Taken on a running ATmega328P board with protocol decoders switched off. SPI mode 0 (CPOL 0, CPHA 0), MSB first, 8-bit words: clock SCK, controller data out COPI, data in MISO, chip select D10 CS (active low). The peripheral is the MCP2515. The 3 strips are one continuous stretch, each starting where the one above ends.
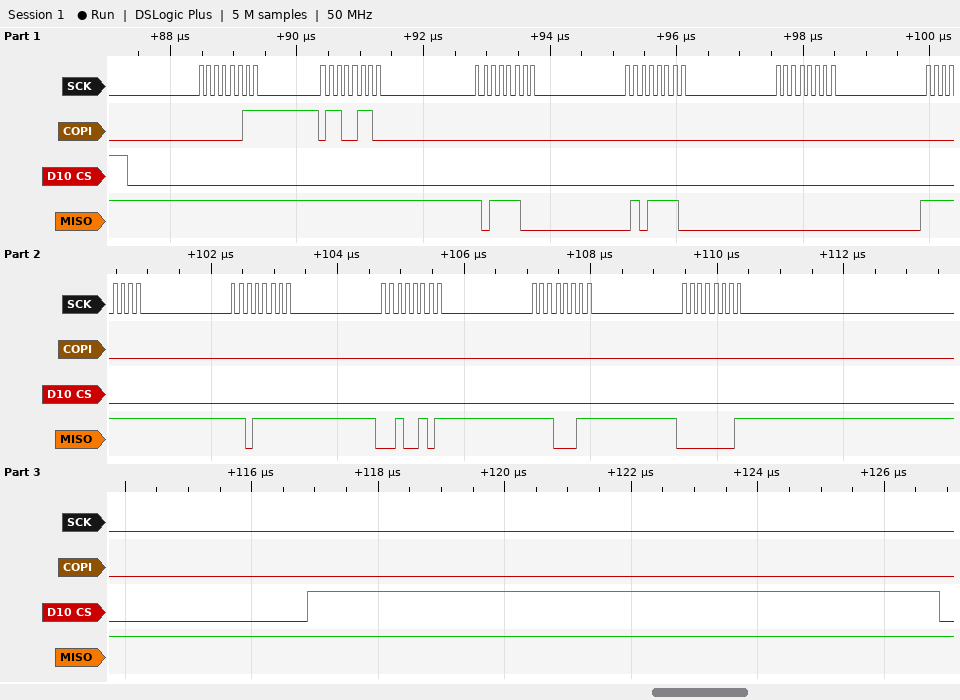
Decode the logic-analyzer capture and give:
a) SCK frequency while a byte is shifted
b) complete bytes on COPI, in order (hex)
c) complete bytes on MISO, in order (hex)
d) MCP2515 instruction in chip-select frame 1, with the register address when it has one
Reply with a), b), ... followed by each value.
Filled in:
a) 8 MHz
b) 0x03 0x66 0x00 0x00 0x00 0x00 0x00 0x00 0x00 0x00
c) 0xFF 0xFF 0xBC 0x5E 0x00 0xFF 0xDF 0x25 0xE3 0x01
d) READ 0x66
